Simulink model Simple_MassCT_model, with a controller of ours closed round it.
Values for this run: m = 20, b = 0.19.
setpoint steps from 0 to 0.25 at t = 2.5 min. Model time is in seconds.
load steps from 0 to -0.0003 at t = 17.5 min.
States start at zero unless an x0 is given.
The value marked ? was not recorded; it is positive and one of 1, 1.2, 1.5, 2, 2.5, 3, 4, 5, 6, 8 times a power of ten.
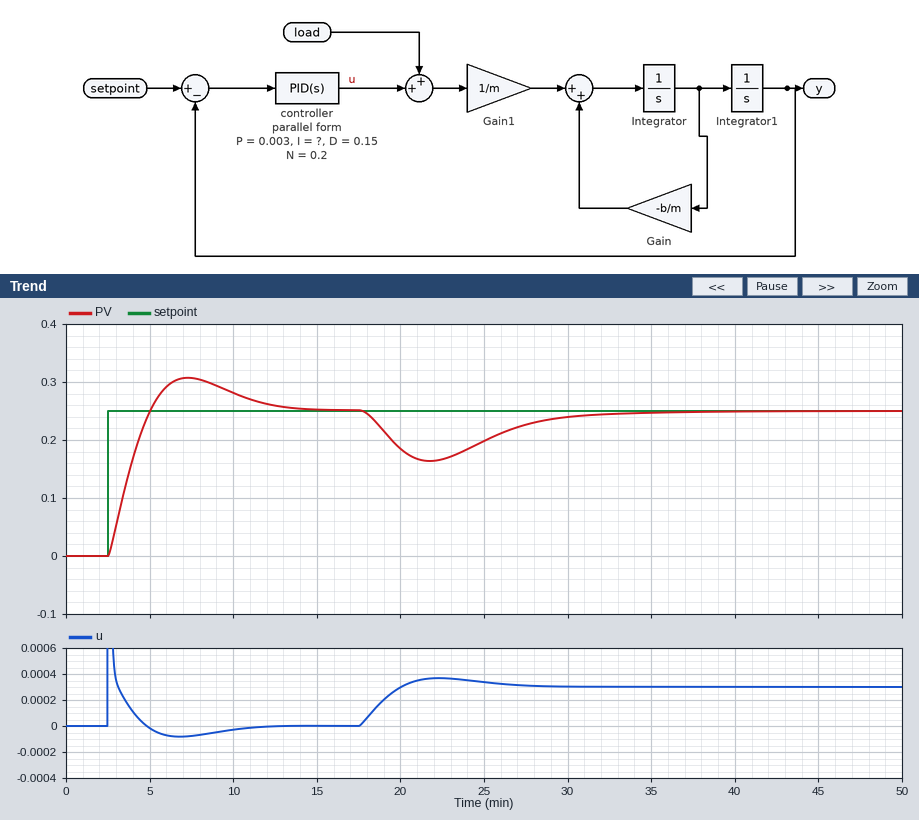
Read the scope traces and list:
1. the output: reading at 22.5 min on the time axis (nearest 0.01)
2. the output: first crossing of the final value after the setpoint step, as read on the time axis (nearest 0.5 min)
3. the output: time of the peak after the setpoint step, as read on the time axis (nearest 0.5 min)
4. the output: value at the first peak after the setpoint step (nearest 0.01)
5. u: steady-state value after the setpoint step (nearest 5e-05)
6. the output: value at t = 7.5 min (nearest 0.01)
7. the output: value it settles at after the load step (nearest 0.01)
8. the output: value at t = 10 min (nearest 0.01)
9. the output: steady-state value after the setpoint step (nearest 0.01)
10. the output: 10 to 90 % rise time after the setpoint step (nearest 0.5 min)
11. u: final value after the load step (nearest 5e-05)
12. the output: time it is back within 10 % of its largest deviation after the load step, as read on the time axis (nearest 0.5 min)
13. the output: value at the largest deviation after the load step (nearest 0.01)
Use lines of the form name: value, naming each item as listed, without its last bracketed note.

the output: reading at 22.5 min on the time axis: 0.17
the output: first crossing of the final value after the setpoint step, as read on the time axis: 5.0 min
the output: time of the peak after the setpoint step, as read on the time axis: 7.5 min
the output: value at the first peak after the setpoint step: 0.31
u: steady-state value after the setpoint step: 0.00000
the output: value at t = 7.5 min: 0.31
the output: value it settles at after the load step: 0.25
the output: value at t = 10 min: 0.28
the output: steady-state value after the setpoint step: 0.25
the output: 10 to 90 % rise time after the setpoint step: 2.0 min
u: final value after the load step: 0.00030
the output: time it is back within 10 % of its largest deviation after the load step, as read on the time axis: 30.5 min
the output: value at the largest deviation after the load step: 0.16
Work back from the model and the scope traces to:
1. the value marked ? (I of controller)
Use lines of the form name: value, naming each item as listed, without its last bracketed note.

the value marked ?: 8e-06
